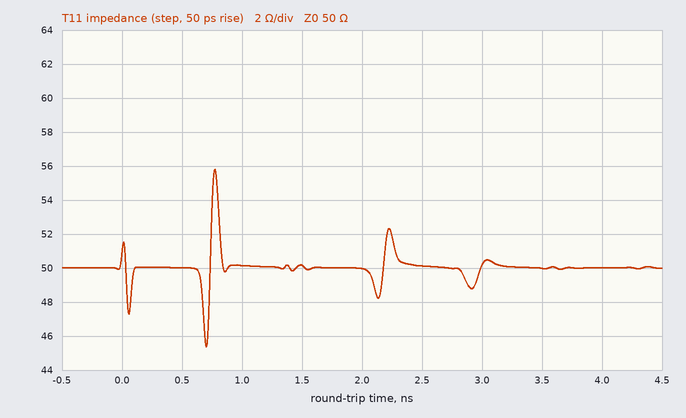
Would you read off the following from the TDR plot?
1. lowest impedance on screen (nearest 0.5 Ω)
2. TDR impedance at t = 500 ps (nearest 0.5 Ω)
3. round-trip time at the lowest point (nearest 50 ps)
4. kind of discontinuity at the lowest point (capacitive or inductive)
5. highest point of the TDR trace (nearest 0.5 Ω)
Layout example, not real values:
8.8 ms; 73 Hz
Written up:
45.5 Ω; 50.0 Ω; 700 ps; capacitive; 56.0 Ω
